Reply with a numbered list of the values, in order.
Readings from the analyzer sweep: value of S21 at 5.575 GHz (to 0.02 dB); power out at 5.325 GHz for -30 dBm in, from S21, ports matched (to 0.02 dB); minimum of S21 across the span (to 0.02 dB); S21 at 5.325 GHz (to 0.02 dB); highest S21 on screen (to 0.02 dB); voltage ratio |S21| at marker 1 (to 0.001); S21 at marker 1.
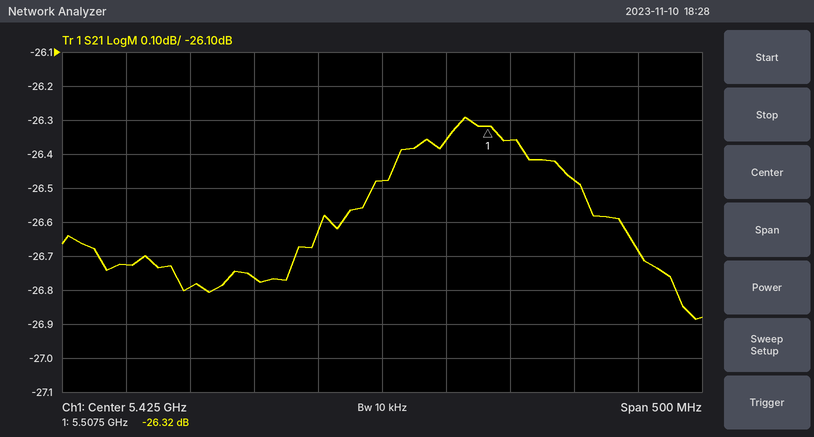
1. -26.48 dB
2. -56.76 dBm
3. -26.88 dB
4. -26.76 dB
5. -26.30 dB
6. 0.048
7. -26.32 dB
